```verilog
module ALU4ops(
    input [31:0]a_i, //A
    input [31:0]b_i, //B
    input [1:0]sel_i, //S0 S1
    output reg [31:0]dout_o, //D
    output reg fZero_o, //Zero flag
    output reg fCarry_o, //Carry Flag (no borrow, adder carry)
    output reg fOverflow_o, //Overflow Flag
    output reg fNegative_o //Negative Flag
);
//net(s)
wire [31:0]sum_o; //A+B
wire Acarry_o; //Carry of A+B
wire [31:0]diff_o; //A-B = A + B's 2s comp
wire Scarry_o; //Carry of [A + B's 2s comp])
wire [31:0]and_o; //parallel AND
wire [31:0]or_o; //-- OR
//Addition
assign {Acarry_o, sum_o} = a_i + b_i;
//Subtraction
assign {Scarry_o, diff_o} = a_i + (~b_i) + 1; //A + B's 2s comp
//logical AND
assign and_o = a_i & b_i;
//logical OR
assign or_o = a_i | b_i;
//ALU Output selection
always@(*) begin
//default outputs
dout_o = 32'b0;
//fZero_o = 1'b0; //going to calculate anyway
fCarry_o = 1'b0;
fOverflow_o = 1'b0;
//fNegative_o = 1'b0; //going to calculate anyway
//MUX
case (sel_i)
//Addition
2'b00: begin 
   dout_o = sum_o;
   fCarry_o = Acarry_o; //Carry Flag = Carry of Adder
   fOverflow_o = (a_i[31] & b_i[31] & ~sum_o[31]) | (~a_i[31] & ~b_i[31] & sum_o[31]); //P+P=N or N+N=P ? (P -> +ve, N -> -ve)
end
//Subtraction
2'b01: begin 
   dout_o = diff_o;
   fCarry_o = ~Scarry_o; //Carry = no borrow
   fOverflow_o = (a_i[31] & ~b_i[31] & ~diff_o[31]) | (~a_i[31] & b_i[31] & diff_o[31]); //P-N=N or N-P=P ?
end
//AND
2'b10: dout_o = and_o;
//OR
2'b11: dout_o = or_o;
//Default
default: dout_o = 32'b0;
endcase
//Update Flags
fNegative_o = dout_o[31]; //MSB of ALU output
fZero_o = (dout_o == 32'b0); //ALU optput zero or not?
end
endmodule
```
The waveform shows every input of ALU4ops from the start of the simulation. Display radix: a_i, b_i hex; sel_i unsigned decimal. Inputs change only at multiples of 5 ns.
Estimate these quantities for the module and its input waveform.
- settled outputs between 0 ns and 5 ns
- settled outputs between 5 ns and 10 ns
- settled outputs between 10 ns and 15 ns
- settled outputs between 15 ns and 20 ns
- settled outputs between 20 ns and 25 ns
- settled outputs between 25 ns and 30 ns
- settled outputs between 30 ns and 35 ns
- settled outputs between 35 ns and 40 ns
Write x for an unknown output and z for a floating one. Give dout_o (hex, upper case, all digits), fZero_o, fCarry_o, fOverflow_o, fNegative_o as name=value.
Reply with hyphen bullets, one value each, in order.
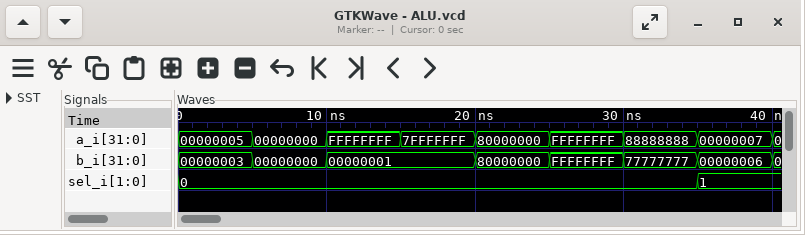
- dout_o=00000008, fZero_o=0, fCarry_o=0, fOverflow_o=0, fNegative_o=0
- dout_o=00000000, fZero_o=1, fCarry_o=0, fOverflow_o=0, fNegative_o=0
- dout_o=00000000, fZero_o=1, fCarry_o=1, fOverflow_o=0, fNegative_o=0
- dout_o=80000000, fZero_o=0, fCarry_o=0, fOverflow_o=1, fNegative_o=1
- dout_o=00000000, fZero_o=1, fCarry_o=1, fOverflow_o=1, fNegative_o=0
- dout_o=FFFFFFFE, fZero_o=0, fCarry_o=1, fOverflow_o=0, fNegative_o=1
- dout_o=FFFFFFFF, fZero_o=0, fCarry_o=0, fOverflow_o=0, fNegative_o=1
- dout_o=00000001, fZero_o=0, fCarry_o=1, fOverflow_o=0, fNegative_o=0
